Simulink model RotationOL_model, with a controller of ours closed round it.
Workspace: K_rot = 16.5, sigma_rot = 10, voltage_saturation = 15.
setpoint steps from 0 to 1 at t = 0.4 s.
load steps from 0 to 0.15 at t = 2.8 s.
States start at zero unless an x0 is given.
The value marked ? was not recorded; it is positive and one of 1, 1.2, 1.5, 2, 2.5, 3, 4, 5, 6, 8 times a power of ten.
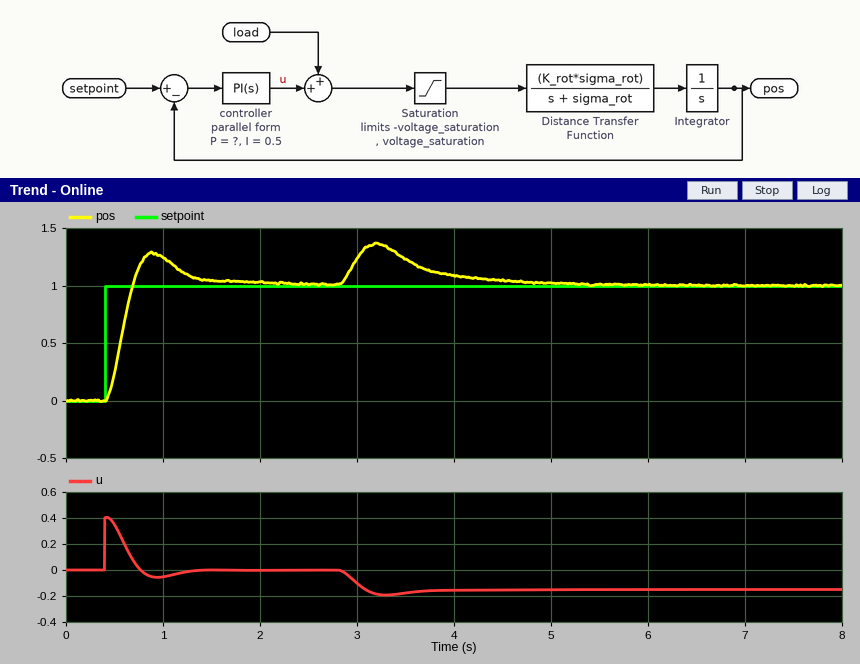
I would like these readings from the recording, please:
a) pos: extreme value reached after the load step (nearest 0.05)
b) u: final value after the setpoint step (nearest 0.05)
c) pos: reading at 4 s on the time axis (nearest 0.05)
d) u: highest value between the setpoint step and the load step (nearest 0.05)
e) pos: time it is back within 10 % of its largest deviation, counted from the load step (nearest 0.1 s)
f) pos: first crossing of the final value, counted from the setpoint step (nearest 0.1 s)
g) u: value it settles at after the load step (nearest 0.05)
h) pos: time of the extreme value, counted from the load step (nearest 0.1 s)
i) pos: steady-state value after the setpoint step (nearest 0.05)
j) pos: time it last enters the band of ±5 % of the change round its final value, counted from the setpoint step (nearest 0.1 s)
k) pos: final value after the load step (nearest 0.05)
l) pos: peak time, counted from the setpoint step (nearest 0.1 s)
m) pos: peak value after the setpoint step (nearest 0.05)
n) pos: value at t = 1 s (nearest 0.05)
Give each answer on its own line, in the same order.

1.35
0.00
1.10
0.40
1.8 s
0.3 s
-0.15
0.4 s
1.00
1.0 s
1.00
0.5 s
1.30
1.25
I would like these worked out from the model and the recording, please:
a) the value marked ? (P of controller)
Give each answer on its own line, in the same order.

0.4
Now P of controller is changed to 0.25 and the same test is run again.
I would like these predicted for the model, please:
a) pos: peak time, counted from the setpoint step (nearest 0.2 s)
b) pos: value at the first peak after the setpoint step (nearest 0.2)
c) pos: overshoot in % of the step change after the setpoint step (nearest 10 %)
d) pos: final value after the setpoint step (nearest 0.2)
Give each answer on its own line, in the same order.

0.6 s
1.4
40 %
1.0
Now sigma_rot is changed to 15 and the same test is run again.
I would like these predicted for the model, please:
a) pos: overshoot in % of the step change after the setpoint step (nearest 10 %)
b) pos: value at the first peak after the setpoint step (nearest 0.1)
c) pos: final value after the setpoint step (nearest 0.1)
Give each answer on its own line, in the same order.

20 %
1.2
1.0
